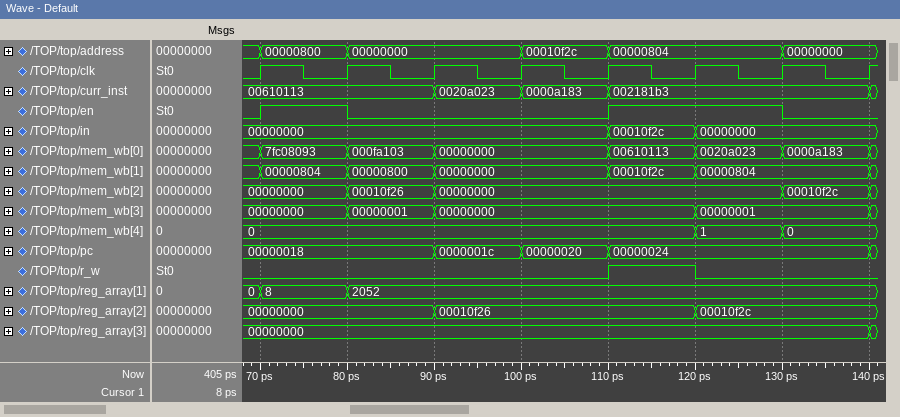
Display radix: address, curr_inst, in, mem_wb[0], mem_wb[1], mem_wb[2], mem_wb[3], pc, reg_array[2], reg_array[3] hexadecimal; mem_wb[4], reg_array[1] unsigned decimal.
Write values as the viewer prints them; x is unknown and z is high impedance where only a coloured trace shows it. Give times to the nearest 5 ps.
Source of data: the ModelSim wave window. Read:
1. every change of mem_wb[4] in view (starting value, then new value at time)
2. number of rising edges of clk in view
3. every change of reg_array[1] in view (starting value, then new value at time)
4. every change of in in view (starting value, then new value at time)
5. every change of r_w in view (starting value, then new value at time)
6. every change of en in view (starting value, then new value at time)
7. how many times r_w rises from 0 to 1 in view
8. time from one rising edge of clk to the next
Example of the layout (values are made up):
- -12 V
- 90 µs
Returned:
- 0, 1 at 120 ps, 0 at 130 ps
- 8
- 0, 8 at 70 ps, 2052 at 80 ps
- 00000000, 00010f2c at 110 ps, 00000000 at 120 ps
- 0, 1 at 110 ps, 0 at 120 ps
- 0, 1 at 70 ps, 0 at 80 ps, 1 at 110 ps, 0 at 130 ps
- 1
- 10 ps
